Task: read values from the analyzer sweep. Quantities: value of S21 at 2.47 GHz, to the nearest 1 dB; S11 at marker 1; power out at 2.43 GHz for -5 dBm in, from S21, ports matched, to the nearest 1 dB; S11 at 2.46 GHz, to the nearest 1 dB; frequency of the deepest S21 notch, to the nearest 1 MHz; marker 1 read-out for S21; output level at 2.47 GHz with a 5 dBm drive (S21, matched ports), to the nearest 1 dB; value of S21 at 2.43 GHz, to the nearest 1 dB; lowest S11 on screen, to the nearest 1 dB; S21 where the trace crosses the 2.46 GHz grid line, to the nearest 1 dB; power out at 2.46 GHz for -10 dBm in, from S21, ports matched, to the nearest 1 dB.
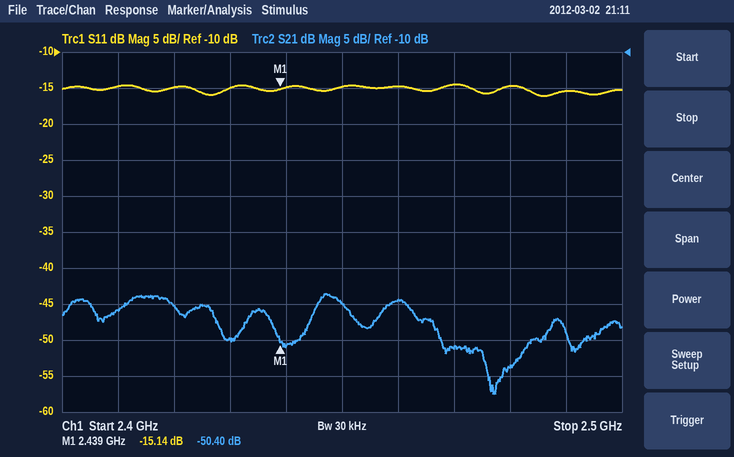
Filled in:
-51 dB
-15.14 dB
-55 dBm
-15 dB
2.477 GHz
-50.40 dB
-46 dBm
-50 dB
-16 dB
-44 dB
-54 dBm
